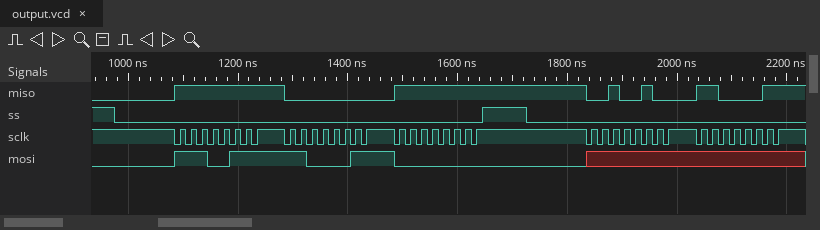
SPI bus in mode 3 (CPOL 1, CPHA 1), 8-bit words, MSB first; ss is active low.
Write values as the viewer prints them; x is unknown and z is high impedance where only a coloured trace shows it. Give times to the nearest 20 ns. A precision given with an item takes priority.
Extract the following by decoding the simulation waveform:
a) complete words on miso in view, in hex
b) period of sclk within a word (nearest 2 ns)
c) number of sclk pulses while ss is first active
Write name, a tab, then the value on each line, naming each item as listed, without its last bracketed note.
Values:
complete words on miso in view, in hex	FF, 00, FF, 24, C3
period of sclk within a word	20 ns
number of sclk pulses while ss is first active	24
